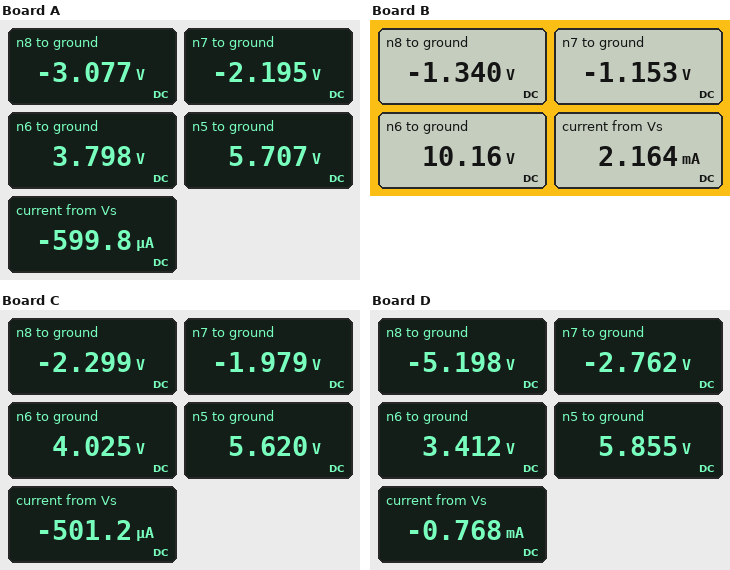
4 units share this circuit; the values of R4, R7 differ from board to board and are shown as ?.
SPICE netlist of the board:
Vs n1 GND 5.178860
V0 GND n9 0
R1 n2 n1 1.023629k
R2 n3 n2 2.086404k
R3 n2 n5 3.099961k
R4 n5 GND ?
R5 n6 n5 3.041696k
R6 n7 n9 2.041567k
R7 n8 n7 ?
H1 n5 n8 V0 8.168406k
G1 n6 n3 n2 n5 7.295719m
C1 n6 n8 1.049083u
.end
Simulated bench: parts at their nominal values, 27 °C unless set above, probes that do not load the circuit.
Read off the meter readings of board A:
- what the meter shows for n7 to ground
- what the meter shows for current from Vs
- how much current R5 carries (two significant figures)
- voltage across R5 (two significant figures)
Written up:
-2.195 V
-599.8 µA
630 µA
1.9 V
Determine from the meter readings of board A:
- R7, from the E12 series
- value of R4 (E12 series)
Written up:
820 Ω
12 kΩ
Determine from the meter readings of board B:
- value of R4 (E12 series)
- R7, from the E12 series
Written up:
1.2 kΩ
330 Ω
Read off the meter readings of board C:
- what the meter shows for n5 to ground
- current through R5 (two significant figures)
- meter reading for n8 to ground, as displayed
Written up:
5.620 V
520 µA
-2.299 V
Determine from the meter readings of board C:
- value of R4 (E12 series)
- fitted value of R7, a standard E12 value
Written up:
12 kΩ
330 Ω
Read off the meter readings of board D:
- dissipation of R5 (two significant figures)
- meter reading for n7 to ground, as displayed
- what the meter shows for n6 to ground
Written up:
2.0 mW
-2.762 V
3.412 V
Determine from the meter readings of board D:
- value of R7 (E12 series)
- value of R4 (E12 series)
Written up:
1.8 kΩ
10 kΩ
